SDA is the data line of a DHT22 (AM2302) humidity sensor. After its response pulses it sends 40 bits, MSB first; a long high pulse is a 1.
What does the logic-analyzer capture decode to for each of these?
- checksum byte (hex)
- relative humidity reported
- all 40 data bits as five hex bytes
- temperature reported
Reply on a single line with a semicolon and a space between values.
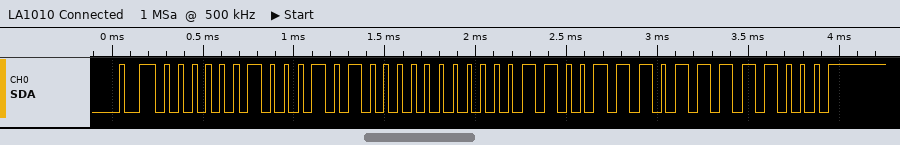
0xF8; 55.2 %; 02 28 00 CE F8; 20.6 °C
